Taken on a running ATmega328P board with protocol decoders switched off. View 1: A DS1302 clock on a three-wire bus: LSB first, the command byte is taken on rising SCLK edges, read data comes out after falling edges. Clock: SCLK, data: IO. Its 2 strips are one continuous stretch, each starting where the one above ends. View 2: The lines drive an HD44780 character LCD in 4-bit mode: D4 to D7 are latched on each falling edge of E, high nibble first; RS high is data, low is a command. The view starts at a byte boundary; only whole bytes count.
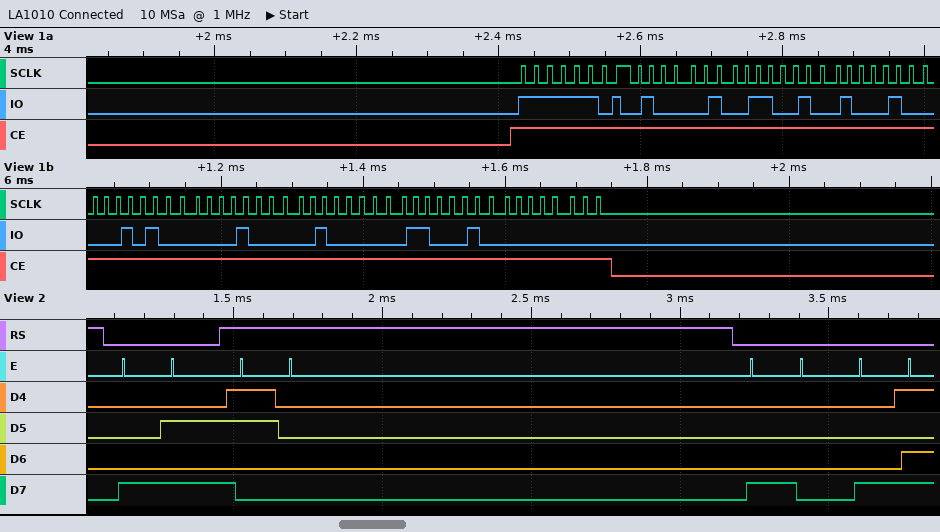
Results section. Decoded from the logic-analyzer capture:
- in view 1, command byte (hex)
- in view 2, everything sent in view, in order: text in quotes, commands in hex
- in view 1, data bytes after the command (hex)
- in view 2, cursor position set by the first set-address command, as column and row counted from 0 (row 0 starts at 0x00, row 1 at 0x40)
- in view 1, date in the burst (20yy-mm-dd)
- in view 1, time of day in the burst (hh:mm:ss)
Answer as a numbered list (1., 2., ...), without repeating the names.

1. 0xBF
2. 0x8A "0" 0x80 0x8D
3. 42 26 11 14 08 02 23 00
4. column 10, row 0
5. 2023-08-14
6. 11:26:42
